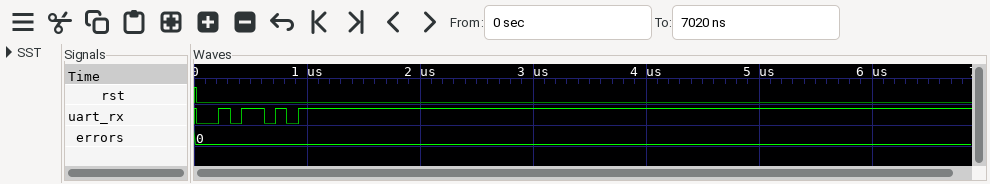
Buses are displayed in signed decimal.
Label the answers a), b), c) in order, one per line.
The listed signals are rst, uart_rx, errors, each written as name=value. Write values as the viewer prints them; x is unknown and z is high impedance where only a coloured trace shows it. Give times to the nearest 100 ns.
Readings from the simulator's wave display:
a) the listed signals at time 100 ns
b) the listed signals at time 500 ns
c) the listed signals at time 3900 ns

a) rst=0, uart_rx=0, errors=0
b) rst=0, uart_rx=1, errors=0
c) rst=0, uart_rx=1, errors=0
